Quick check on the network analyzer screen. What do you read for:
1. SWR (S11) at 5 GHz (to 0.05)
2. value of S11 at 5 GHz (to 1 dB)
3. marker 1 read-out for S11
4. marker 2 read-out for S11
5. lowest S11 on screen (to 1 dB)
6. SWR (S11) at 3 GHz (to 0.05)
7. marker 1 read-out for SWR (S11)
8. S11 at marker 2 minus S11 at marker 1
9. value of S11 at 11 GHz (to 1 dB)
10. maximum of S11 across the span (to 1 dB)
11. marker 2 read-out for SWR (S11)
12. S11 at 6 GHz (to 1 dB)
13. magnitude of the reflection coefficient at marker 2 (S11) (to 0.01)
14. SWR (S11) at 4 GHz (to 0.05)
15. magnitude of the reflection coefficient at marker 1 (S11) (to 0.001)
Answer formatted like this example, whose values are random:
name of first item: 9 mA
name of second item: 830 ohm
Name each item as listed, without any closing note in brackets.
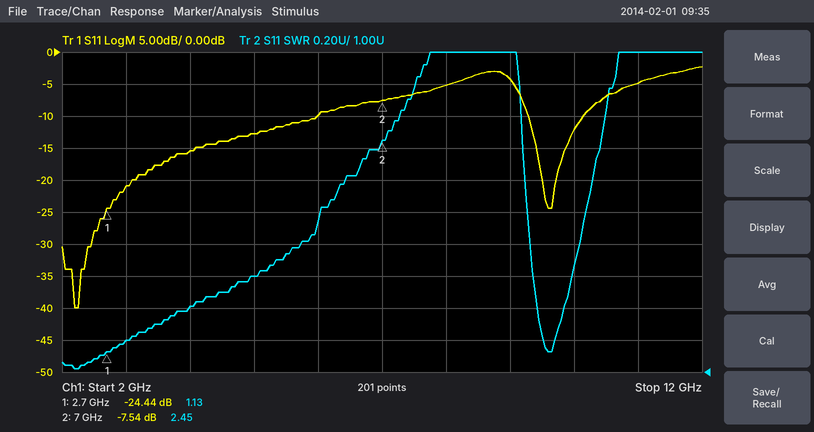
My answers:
SWR (S11) at 5 GHz: 1.60
value of S11 at 5 GHz: -13 dB
marker 1 read-out for S11: -24.44 dB
marker 2 read-out for S11: -7.54 dB
lowest S11 on screen: -40 dB
SWR (S11) at 3 GHz: 1.20
marker 1 read-out for SWR: 1.13
S11 at marker 2 minus S11 at marker 1: 16.90 dB
value of S11 at 11 GHz: -5 dB
maximum of S11 across the span: -2 dB
marker 2 read-out for SWR: 2.45
S11 at 6 GHz: -10 dB
magnitude of the reflection coefficient at marker 2 (S11): 0.42
SWR (S11) at 4 GHz: 1.40
magnitude of the reflection coefficient at marker 1 (S11): 0.060
